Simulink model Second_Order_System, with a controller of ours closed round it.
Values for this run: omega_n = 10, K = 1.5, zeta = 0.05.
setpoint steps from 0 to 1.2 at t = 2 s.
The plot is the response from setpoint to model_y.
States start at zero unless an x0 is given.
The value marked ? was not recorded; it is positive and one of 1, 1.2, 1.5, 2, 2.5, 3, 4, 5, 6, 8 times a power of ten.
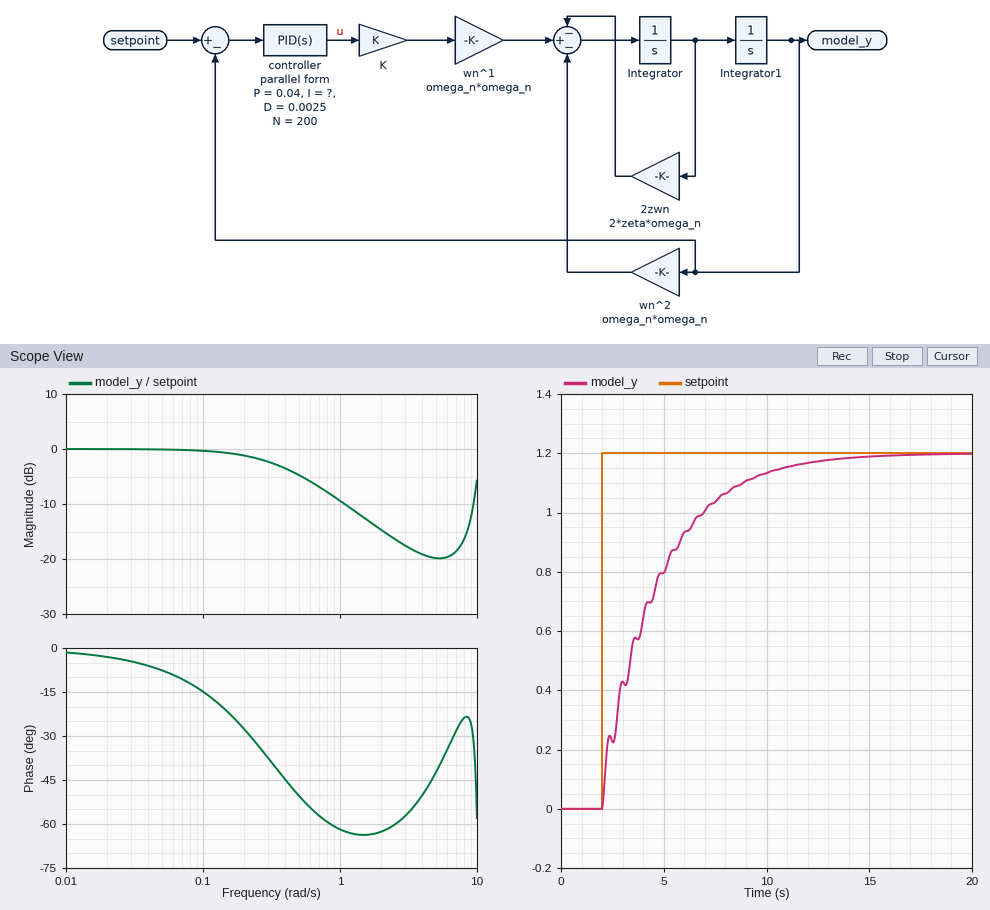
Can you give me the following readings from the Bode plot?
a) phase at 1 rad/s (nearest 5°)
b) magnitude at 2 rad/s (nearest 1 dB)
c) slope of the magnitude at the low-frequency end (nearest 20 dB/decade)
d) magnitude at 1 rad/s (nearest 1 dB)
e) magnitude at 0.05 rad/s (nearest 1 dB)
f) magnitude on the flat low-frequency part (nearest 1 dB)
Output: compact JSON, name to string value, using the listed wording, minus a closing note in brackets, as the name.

{"phase at 1 rad/s": "-60°", "magnitude at 2 rad/s": "-15 dB", "slope of the magnitude at the low-frequency end": "0 dB/decade", "magnitude at 1 rad/s": "-9 dB", "magnitude at 0.05 rad/s": "0 dB", "magnitude on the flat low-frequency part": "0 dB"}
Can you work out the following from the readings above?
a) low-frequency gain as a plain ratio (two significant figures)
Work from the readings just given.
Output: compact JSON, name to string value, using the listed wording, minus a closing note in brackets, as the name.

{"low-frequency gain as a plain ratio": "1.0"}
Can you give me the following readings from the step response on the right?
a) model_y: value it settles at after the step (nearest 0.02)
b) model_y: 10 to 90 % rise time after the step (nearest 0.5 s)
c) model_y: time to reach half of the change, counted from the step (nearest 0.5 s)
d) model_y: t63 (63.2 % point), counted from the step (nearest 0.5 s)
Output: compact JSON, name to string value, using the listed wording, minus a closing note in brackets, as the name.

{"model_y: value it settles at after the step": "1.20", "model_y: 10 to 90 % rise time after the step": "6.0 s", "model_y: time to reach half of the change, counted from the step": "2.0 s", "model_y: t63 (63.2 % point), counted from the step": "2.5 s"}
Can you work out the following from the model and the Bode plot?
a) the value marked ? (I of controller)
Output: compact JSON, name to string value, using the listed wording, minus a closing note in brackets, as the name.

{"the value marked ?": "0.25"}
